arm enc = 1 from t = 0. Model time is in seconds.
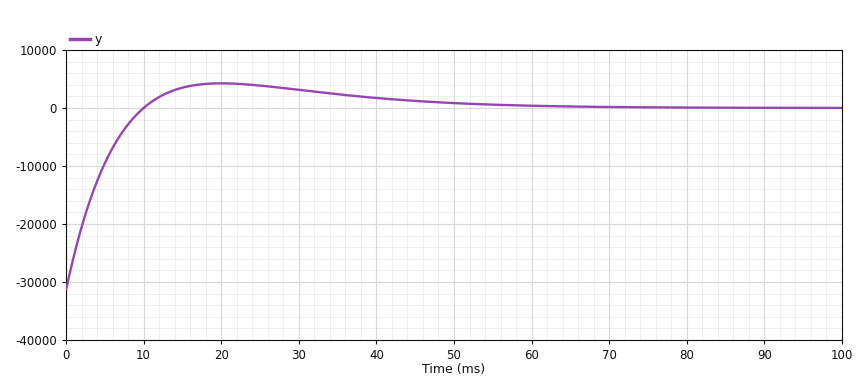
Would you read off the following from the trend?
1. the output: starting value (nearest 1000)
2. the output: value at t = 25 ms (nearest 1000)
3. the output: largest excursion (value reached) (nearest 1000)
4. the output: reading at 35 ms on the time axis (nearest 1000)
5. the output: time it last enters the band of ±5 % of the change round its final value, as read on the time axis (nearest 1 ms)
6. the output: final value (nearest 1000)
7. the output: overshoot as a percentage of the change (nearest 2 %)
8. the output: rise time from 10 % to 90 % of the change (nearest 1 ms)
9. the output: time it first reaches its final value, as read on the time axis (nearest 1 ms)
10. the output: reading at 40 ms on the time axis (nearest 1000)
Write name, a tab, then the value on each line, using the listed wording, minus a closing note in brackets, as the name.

the output: starting value	-31000
the output: value at t = 25 ms	4000
the output: largest excursion (value reached)	4000
the output: reading at 35 ms on the time axis	2000
the output: time it last enters the band of ±5 % of the change round its final value, as read on the time axis	41 ms
the output: final value	0
the output: overshoot as a percentage of the change	14 %
the output: rise time from 10 % to 90 % of the change	7 ms
the output: time it first reaches its final value, as read on the time axis	10 ms
the output: reading at 40 ms on the time axis	2000
